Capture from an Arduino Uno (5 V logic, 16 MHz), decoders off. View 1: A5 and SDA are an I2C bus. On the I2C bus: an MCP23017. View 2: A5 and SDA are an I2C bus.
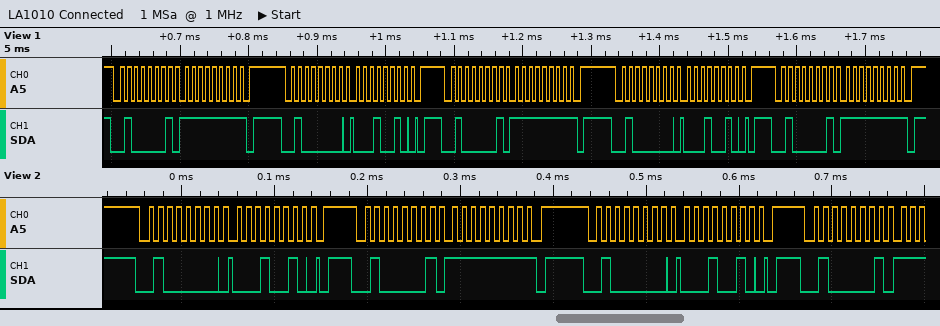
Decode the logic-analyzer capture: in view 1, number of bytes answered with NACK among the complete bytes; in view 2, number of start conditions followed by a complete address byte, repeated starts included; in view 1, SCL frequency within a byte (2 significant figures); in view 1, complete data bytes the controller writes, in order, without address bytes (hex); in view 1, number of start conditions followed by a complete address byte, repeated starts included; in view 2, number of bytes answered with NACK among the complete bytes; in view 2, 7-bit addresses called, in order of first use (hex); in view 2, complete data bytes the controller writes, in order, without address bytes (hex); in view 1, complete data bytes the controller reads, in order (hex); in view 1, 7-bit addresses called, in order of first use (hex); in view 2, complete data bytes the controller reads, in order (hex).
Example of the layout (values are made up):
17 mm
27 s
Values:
3
4
100 kHz
12 12
5
1
0x20
12 12
FF FF FF
0x20
FF
